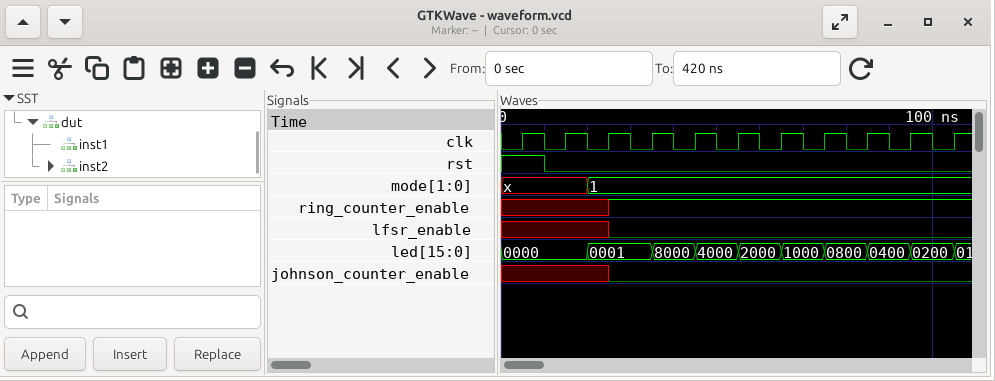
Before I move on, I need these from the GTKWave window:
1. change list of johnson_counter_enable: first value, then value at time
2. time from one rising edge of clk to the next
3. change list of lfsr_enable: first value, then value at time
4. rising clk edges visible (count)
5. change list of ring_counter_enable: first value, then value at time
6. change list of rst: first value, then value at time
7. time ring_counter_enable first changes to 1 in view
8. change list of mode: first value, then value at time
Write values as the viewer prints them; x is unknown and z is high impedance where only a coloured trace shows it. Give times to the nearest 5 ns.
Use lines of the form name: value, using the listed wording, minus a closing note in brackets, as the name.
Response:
change list of johnson_counter_enable: first value, then value at time: x, 0 at 25 ns
time from one rising edge of clk to the next: 10 ns
change list of lfsr_enable: first value, then value at time: x, 0 at 25 ns
rising clk edges visible: 11
change list of ring_counter_enable: first value, then value at time: x, 1 at 25 ns
change list of rst: first value, then value at time: 1, 0 at 10 ns
time ring_counter_enable first changes to 1 in view: 25 ns
change list of mode: first value, then value at time: x, 1 at 20 ns
